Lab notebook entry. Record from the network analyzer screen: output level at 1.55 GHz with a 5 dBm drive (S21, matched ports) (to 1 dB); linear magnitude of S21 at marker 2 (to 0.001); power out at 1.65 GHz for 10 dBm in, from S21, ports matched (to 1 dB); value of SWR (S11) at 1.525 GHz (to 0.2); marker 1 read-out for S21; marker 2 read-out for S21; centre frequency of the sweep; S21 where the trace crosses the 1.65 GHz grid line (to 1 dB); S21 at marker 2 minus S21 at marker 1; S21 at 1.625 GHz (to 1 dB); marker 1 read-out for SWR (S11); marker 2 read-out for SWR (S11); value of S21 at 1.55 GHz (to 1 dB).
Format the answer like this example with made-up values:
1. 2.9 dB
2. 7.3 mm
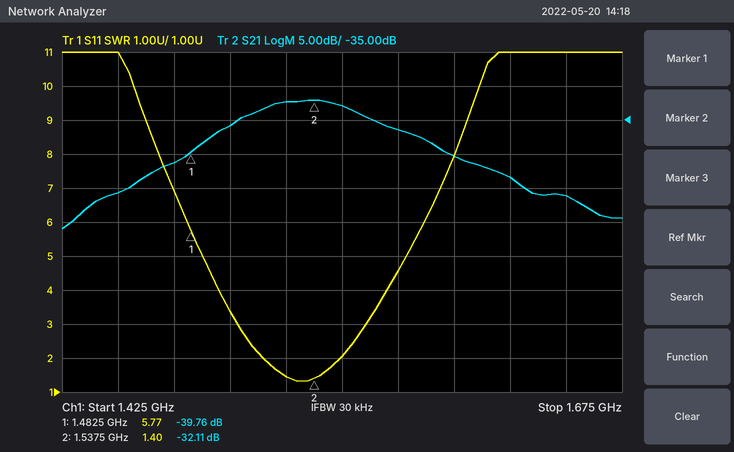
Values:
1. -28 dBm
2. 0.025
3. -36 dBm
4. 1.4
5. -39.76 dB
6. -32.11 dB
7. 1.55 GHz
8. -46 dB
9. 7.65 dB
10. -43 dB
11. 5.77
12. 1.40
13. -33 dB
